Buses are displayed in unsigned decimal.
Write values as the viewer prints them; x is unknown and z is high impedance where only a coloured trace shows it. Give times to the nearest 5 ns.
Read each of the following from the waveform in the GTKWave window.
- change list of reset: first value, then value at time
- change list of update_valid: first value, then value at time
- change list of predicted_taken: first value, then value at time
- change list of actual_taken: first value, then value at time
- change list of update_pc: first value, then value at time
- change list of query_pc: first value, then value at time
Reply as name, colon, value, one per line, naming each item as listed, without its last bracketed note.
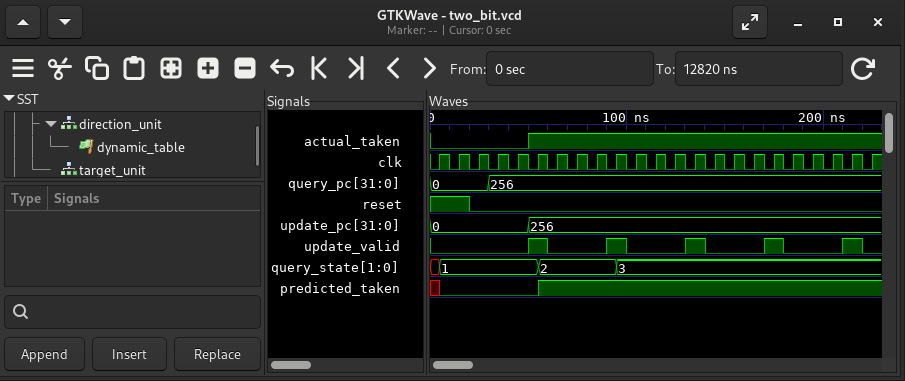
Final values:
change list of reset: first value, then value at time: 1, 0 at 20 ns
change list of update_valid: first value, then value at time: 0, 1 at 50 ns, 0 at 60 ns, 1 at 90 ns, 0 at 100 ns, 1 at 130 ns, 0 at 140 ns, 1 at 170 ns, 0 at 180 ns, 1 at 210 ns, 0 at 220 ns
change list of predicted_taken: first value, then value at time: x, 0 at 5 ns, 1 at 55 ns
change list of actual_taken: first value, then value at time: 0, 1 at 50 ns
change list of update_pc: first value, then value at time: 0, 256 at 50 ns
change list of query_pc: first value, then value at time: 0, 256 at 30 ns
